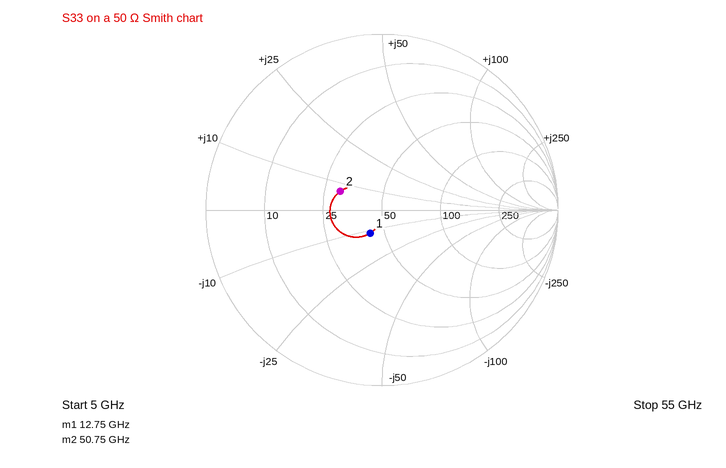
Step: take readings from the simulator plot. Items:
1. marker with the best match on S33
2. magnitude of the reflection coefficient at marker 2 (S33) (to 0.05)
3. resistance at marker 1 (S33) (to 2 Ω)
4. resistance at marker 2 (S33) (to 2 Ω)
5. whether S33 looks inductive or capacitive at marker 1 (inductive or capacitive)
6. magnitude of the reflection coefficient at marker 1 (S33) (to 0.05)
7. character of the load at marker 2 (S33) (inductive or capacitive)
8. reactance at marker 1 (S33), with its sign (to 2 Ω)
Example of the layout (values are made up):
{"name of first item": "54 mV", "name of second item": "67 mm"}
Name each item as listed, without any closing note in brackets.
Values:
{"marker with the best match on S33": "marker 1", "magnitude of the reflection coefficient at marker 2 (S33)": "0.25", "resistance at marker 1 (S33)": "42 Ω", "resistance at marker 2 (S33)": "30 Ω", "whether S33 looks inductive or capacitive at marker 1": "capacitive", "magnitude of the reflection coefficient at marker 1 (S33)": "0.15", "character of the load at marker 2 (S33)": "inductive", "reactance at marker 1 (S33), with its sign": "-12 Ω"}
